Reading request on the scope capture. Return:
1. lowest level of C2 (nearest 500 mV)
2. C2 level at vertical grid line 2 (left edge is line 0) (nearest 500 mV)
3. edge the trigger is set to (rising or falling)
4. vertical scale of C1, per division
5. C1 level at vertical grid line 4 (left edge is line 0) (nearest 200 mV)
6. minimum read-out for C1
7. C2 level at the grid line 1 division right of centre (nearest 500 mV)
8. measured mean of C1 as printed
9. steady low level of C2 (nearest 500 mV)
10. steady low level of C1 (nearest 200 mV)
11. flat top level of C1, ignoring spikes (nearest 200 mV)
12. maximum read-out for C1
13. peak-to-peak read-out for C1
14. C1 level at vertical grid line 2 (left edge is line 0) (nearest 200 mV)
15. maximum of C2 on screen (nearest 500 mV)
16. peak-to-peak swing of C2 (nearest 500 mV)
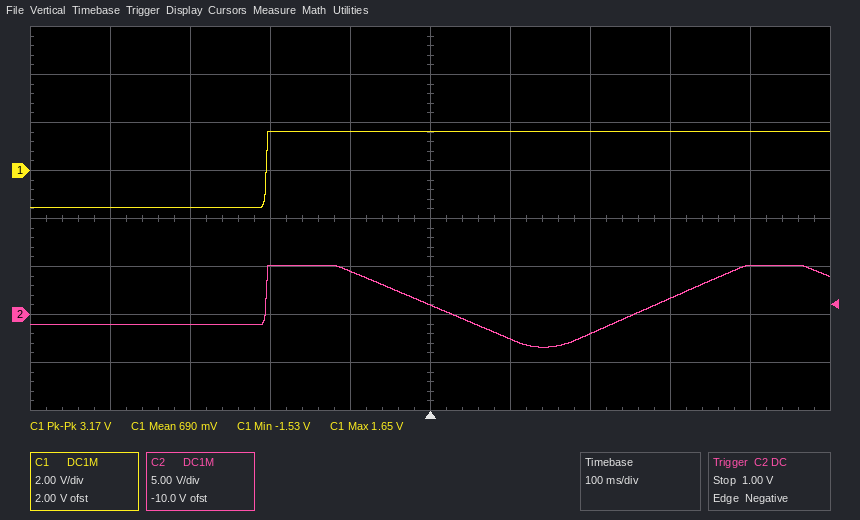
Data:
-3.5 V
-1.0 V
falling
2 V
1.6 V
-1.53 V
-2.5 V
690 mV
-1.0 V
-1.6 V
1.6 V
1.65 V
3.17 V
-1.6 V
5.0 V
8.5 V
